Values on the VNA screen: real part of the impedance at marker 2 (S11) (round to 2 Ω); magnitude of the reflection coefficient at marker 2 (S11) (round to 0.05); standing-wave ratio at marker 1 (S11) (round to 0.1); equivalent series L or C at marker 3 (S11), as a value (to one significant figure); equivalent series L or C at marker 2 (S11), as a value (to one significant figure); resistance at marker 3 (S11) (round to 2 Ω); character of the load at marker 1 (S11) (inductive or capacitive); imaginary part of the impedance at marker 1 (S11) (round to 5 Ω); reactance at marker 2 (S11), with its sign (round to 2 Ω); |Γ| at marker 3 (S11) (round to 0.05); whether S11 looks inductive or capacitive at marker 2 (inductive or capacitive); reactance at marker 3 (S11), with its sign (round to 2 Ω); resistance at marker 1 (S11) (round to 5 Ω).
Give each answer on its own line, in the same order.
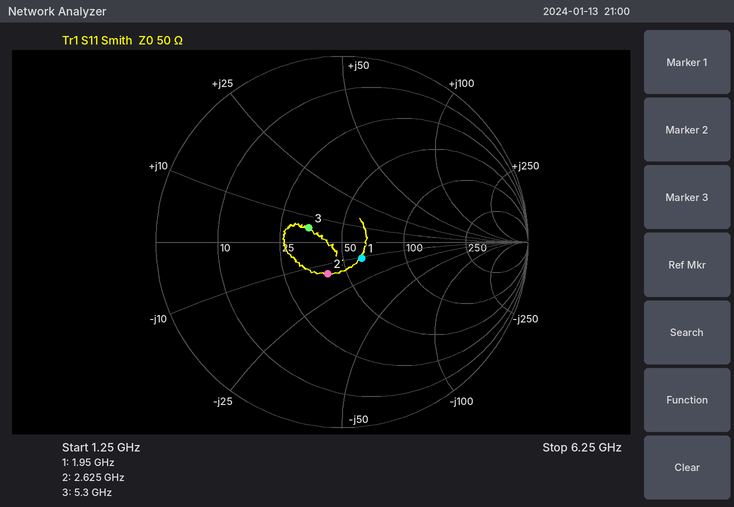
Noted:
40 Ω
0.20
1.3
200 pH
4 pF
34 Ω
capacitive
-10 Ω
-14 Ω
0.20
capacitive
+6 Ω
60 Ω
